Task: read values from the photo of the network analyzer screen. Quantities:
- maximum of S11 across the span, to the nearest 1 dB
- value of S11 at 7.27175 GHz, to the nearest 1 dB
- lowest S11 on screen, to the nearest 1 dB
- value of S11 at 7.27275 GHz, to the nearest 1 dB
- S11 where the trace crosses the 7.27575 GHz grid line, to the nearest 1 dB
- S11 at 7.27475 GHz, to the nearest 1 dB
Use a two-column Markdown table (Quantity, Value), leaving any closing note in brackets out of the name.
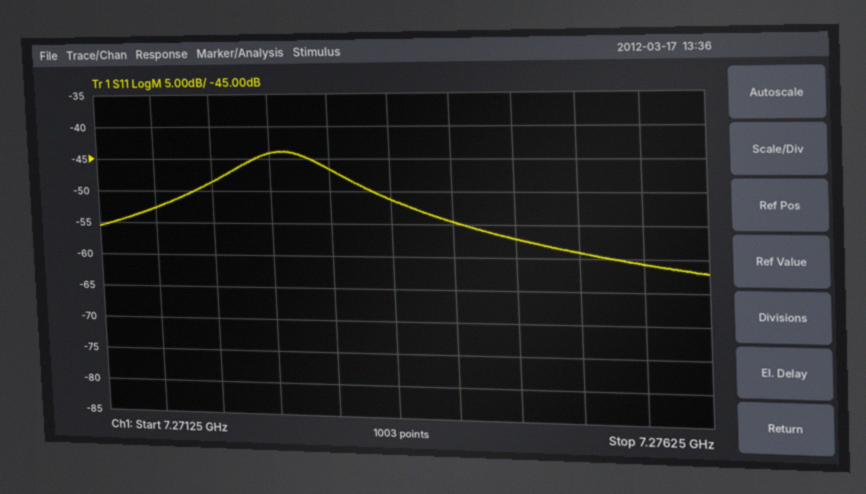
| Quantity | Value |
|---|---|
| maximum of S11 across the span, to the nearest 1 dB | -44 dB |
| value of S11 at 7.27175 GHz, to the nearest 1 dB | -53 dB |
| lowest S11 on screen, to the nearest 1 dB | -62 dB |
| value of S11 at 7.27275 GHz, to the nearest 1 dB | -44 dB |
| S11 where the trace crosses the 7.27575 GHz grid line, to the nearest 1 dB | -61 dB |
| S11 at 7.27475 GHz, to the nearest 1 dB | -57 dB |
